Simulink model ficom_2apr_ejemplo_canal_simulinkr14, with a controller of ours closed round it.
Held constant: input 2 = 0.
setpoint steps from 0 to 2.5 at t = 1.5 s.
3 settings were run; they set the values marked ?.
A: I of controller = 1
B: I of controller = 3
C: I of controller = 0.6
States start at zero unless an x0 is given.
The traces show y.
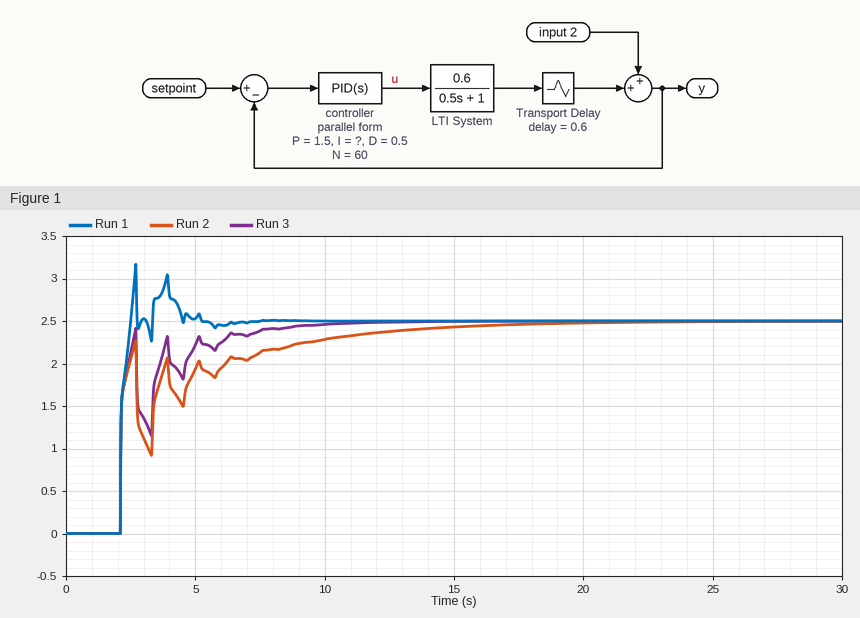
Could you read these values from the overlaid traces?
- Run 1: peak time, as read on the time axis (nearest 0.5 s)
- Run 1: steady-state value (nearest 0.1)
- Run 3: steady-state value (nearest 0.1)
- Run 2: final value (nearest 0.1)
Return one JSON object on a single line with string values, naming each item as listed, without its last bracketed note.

{"Run 1: peak time, as read on the time axis": "2.5 s", "Run 1: steady-state value": "2.5", "Run 3: steady-state value": "2.5", "Run 2: final value": "2.5"}
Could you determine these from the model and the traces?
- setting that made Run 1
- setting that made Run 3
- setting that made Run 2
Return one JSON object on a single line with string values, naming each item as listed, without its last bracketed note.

{"setting that made Run 1": "B", "setting that made Run 3": "A", "setting that made Run 2": "C"}
